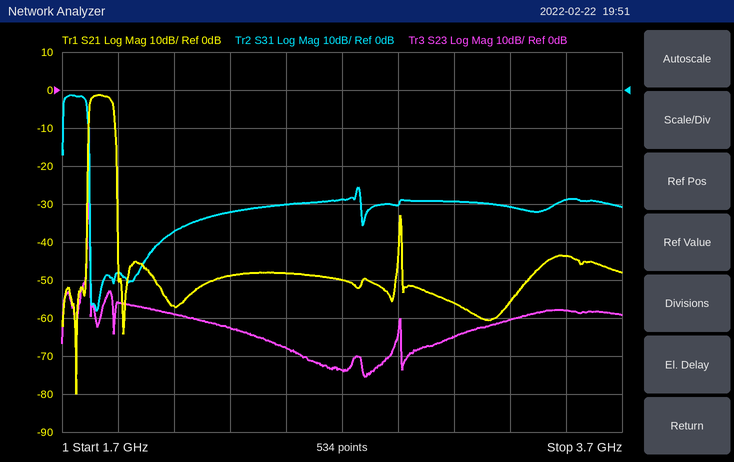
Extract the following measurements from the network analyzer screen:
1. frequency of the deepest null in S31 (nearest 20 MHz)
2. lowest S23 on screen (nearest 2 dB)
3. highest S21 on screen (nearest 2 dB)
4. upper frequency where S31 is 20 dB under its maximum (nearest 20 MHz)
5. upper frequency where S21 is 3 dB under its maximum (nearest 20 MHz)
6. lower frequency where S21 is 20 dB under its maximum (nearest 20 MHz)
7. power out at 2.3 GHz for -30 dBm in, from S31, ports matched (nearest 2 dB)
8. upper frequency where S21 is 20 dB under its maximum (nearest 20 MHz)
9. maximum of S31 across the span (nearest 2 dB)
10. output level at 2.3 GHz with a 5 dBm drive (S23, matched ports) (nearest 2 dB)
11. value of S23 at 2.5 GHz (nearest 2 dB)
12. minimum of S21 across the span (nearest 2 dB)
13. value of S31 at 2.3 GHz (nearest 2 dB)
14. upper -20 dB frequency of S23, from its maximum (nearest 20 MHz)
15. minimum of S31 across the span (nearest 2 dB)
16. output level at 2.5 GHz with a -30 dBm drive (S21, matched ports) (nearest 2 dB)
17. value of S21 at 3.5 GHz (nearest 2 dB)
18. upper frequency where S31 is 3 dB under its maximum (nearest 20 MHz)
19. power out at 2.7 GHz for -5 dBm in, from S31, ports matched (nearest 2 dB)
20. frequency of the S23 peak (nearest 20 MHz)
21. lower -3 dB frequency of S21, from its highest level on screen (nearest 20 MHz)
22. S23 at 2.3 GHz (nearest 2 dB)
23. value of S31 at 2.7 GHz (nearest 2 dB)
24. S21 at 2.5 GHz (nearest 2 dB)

1.82 GHz
-76 dB
-2 dB
1.80 GHz
1.88 GHz
1.80 GHz
-62 dBm
1.90 GHz
-2 dB
-58 dBm
-68 dB
-80 dB
-32 dB
1.80 GHz
-58 dB
-78 dBm
-44 dB
1.78 GHz
-34 dBm
1.80 GHz
1.80 GHz
-62 dB
-28 dB
-48 dB
